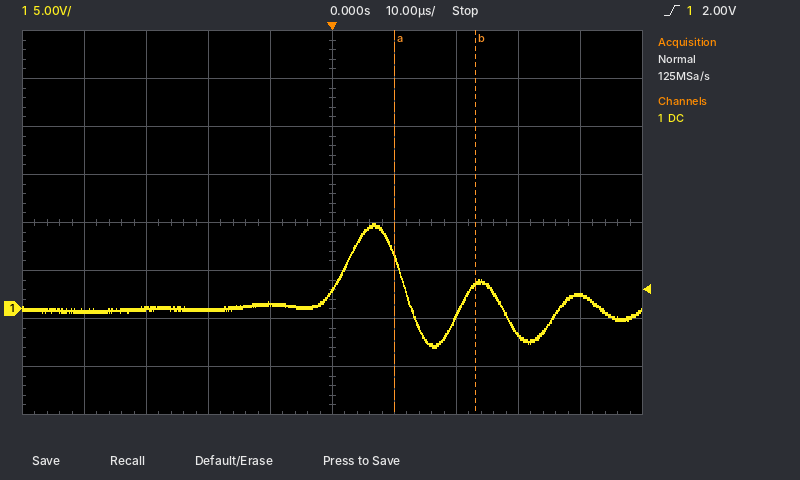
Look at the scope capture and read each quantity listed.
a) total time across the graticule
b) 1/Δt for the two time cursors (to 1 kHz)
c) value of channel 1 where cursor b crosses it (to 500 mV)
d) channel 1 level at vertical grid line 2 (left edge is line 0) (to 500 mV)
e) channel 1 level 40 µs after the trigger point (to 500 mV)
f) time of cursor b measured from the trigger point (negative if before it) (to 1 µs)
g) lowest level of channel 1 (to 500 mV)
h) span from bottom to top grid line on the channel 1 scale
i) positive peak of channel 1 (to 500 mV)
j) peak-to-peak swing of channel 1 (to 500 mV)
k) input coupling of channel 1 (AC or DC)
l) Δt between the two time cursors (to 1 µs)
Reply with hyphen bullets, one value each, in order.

- 100 µs
- 77 kHz
- 2.5 V
- 0.0 V
- 1.5 V
- +23 µs
- -4.0 V
- 40 V
- 9.0 V
- 13.0 V
- DC
- 13 µs
